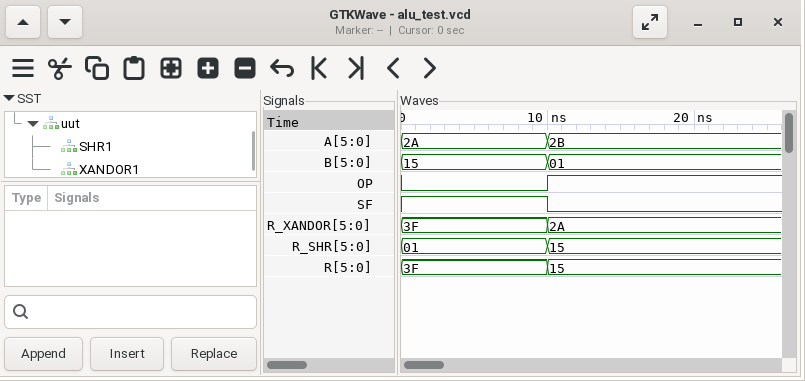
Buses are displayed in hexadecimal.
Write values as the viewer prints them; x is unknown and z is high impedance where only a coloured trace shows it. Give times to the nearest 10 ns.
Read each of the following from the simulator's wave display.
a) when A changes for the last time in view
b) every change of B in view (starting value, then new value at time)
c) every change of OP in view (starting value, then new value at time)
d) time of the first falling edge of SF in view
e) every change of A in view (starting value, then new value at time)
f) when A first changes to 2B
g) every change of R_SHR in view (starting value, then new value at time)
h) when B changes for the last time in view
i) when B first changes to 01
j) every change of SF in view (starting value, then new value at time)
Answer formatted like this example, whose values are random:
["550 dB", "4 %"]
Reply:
["10 ns", "15, 01 at 10 ns", "0, 1 at 10 ns", "10 ns", "2A, 2B at 10 ns", "10 ns", "01, 15 at 10 ns", "10 ns", "10 ns", "1, 0 at 10 ns"]
